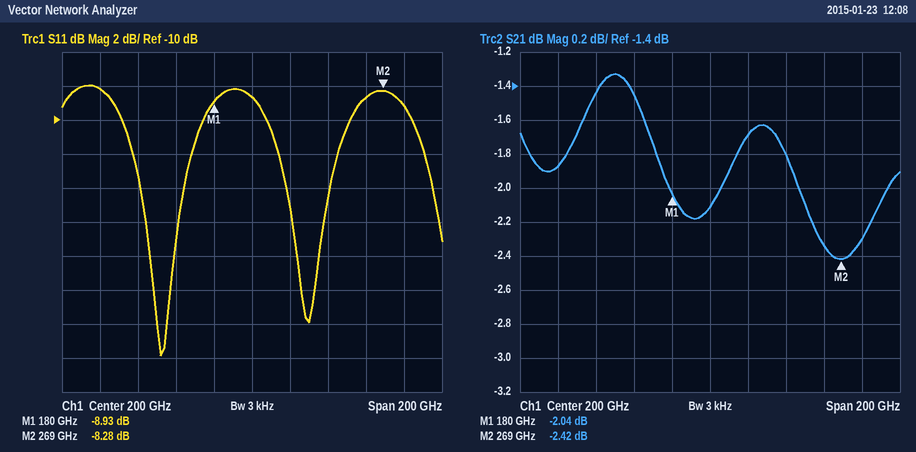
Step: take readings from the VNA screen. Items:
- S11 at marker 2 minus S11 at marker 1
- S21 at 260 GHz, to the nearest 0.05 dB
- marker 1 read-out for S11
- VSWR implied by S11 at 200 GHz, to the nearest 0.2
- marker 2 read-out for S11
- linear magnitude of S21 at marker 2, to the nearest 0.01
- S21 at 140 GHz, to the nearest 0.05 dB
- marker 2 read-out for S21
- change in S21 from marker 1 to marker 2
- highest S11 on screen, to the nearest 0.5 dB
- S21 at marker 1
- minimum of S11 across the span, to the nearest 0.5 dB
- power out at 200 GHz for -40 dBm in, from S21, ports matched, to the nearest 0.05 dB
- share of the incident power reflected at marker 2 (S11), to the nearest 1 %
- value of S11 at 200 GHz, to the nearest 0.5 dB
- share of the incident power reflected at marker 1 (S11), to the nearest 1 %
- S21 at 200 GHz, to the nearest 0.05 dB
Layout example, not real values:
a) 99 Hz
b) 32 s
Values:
a) 0.65 dB
b) -2.35 dB
c) -8.93 dB
d) 2.2
e) -8.28 dB
f) 0.76
g) -1.45 dB
h) -2.42 dB
i) -0.38 dB
j) -8.0 dB
k) -2.04 dB
l) -24.0 dB
m) -42.10 dBm
n) 15 %
o) -8.5 dB
p) 13 %
q) -2.10 dB
